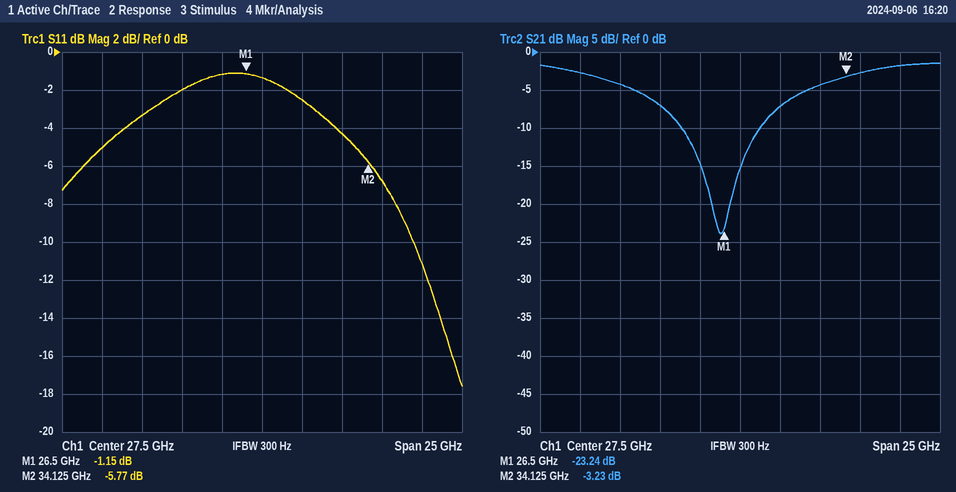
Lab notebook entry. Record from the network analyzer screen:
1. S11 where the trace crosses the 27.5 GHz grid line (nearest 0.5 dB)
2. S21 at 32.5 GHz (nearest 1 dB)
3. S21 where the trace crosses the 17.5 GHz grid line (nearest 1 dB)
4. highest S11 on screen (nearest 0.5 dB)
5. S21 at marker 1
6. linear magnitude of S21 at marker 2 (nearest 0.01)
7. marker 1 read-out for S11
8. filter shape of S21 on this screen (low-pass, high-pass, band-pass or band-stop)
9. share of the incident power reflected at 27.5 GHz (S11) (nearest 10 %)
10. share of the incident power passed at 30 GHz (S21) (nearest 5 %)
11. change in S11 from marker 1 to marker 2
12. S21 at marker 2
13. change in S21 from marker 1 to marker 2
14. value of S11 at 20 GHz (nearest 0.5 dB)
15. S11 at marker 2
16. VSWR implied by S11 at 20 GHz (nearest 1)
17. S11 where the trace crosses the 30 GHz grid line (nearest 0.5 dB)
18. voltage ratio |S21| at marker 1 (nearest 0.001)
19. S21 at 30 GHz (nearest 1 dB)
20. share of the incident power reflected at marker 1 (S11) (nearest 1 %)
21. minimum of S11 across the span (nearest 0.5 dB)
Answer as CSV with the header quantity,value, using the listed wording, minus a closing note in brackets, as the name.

quantity,value
S11 where the trace crosses the 27.5 GHz grid line,-1.5 dB
S21 at 32.5 GHz,-4 dB
S21 where the trace crosses the 17.5 GHz grid line,-3 dB
highest S11 on screen,-1.0 dB
S21 at marker 1,-23.24 dB
linear magnitude of S21 at marker 2,0.69
marker 1 read-out for S11,-1.15 dB
filter shape of S21 on this screen,band-stop
share of the incident power reflected at 27.5 GHz (S11),70 %
share of the incident power passed at 30 GHz (S21),20 %
change in S11 from marker 1 to marker 2,-4.62 dB
S21 at marker 2,-3.23 dB
change in S21 from marker 1 to marker 2,20.01 dB
value of S11 at 20 GHz,-3.5 dB
S11 at marker 2,-5.77 dB
VSWR implied by S11 at 20 GHz,5
S11 where the trace crosses the 30 GHz grid line,-2.5 dB
voltage ratio |S21| at marker 1,0.069
S21 at 30 GHz,-7 dB
share of the incident power reflected at marker 1 (S11),77 %
minimum of S11 across the span,-17.5 dB
